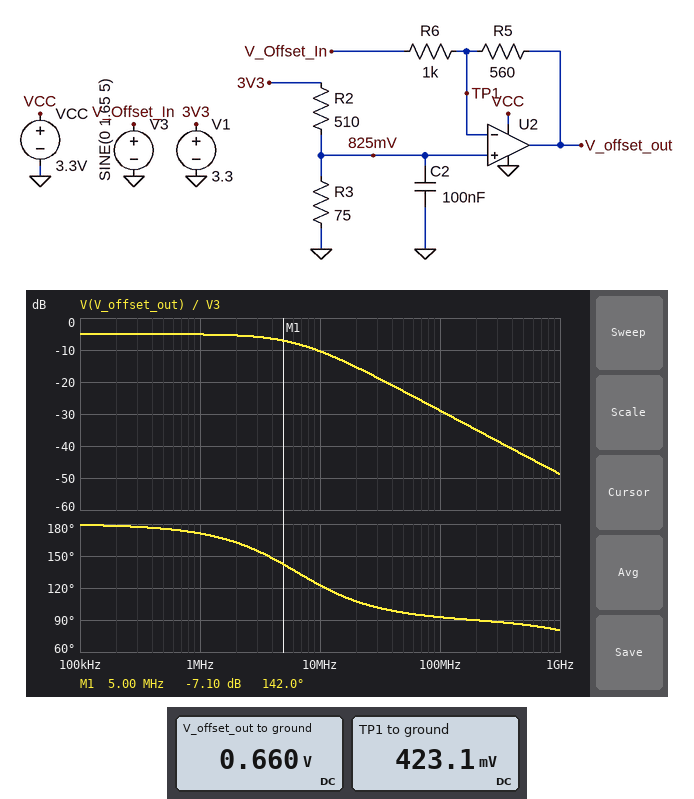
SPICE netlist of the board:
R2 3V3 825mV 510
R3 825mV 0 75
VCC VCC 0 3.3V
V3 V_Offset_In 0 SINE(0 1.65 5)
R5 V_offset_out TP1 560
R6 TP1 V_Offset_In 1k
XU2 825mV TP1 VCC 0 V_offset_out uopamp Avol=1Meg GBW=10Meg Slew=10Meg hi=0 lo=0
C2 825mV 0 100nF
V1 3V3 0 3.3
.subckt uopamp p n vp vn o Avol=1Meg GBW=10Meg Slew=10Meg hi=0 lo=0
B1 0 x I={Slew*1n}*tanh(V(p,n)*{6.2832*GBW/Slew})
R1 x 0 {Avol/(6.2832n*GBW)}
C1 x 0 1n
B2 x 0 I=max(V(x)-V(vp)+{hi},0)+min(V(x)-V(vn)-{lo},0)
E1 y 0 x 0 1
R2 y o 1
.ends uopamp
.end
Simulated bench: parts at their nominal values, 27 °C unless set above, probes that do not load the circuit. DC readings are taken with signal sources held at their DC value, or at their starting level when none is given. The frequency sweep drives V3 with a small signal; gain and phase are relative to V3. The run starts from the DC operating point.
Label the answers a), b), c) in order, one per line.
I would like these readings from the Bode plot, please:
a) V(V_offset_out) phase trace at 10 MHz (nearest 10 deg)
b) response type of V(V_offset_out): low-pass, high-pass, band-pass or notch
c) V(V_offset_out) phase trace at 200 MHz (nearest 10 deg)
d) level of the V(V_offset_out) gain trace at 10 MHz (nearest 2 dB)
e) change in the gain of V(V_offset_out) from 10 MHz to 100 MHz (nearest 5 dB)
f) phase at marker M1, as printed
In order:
a) 120 deg
b) low-pass
c) 90 deg
d) -10 dB
e) -20 dB
f) 142.0 deg
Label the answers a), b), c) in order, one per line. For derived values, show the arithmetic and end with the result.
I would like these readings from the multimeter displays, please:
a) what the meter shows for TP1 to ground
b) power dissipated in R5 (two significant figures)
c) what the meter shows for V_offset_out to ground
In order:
a) 423.1 mV
b) (660 mV - 423.1 mV)^2 / 560 Ω = 100 µW
c) 0.660 V
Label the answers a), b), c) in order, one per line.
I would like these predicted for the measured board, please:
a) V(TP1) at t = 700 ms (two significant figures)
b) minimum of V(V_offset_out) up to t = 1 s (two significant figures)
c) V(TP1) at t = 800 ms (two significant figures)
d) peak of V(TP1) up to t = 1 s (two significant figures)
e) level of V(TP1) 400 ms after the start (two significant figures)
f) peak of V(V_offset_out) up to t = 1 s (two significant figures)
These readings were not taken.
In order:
a) 420 mV
b) -6.7 mV
c) 420 mV
d) 590 mV
e) 420 mV
f) 1.6 V
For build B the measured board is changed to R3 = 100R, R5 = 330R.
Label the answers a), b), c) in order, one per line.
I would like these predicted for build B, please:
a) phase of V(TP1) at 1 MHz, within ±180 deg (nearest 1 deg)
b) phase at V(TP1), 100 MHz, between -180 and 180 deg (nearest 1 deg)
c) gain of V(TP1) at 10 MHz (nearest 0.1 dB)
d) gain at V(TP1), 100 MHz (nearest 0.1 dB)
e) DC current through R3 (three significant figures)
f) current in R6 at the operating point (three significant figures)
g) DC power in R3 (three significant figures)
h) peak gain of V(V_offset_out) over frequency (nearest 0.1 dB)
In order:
a) 82 deg
b) 4 deg
c) -14.0 dB
d) -12.1 dB
e) 5.41 mA
f) 541 µA
g) 2.93 mW
h) -9.6 dB
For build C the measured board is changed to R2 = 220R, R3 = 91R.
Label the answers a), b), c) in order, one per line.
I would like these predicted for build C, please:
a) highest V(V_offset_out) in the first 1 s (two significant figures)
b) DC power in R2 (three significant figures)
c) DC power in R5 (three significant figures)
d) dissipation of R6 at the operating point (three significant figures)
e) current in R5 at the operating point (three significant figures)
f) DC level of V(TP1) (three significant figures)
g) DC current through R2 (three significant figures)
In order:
a) 2.4 V
b) 24.8 mW
c) 522 µW
d) 932 µW
e) 966 µA
f) 966 mV
g) 10.6 mA
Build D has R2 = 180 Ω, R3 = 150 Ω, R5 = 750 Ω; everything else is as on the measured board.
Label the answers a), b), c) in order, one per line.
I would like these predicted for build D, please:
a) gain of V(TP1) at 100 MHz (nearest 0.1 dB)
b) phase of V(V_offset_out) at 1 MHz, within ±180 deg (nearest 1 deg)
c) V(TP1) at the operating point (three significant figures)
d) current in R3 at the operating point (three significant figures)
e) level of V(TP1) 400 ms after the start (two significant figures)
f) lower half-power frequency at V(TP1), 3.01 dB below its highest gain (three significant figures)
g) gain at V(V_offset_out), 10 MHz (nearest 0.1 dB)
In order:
a) -7.4 dB
b) 170 deg
c) 1.50 V
d) 10.0 mA
e) 1.5 V
f) 5.71 MHz
g) -8.6 dB
